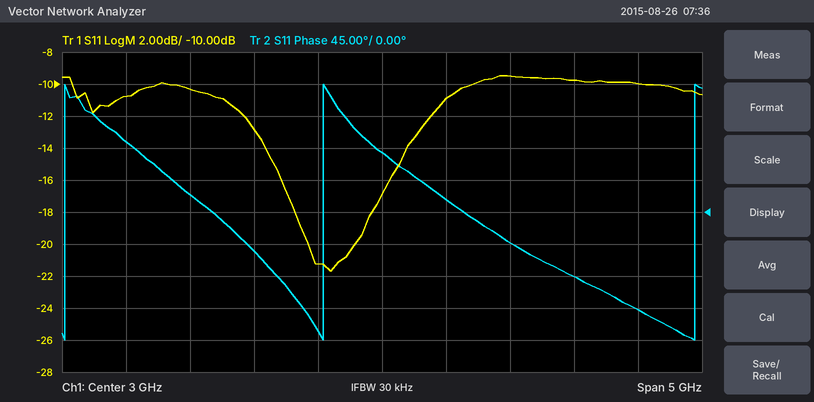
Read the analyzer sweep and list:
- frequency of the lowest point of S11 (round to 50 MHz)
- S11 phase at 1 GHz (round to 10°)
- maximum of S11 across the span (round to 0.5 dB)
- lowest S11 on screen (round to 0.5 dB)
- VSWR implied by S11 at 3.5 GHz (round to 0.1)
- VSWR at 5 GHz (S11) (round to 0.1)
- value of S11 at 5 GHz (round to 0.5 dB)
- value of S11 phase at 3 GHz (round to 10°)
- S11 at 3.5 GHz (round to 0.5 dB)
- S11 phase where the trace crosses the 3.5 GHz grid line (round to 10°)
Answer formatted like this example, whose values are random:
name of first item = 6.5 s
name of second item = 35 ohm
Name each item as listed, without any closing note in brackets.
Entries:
frequency of the lowest point of S11 = 2.60 GHz
S11 phase at 1 GHz = 100°
maximum of S11 across the span = -9.5 dB
lowest S11 on screen = -21.5 dB
VSWR implied by S11 at 3.5 GHz = 1.8
VSWR at 5 GHz (S11) = 1.9
value of S11 at 5 GHz = -10.0 dB
value of S11 phase at 3 GHz = 80°
S11 at 3.5 GHz = -11.0 dB
S11 phase where the trace crosses the 3.5 GHz grid line = 20°
